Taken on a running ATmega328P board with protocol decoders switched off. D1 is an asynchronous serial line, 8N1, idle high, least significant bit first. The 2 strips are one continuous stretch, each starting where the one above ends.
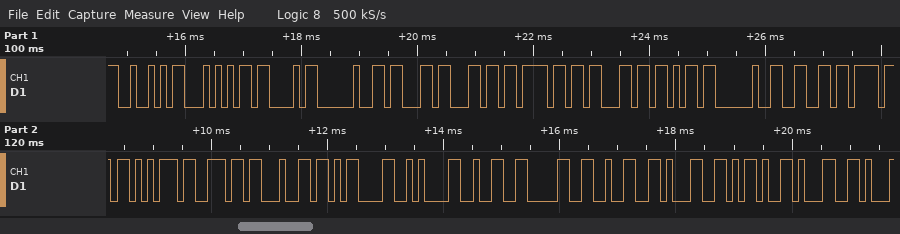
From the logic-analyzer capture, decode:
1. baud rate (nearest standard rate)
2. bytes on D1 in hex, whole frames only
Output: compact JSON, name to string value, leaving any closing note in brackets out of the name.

{"baud rate": "9600 baud", "bytes on D1 in hex, whole frames only": "0x52 0x54 0x43 0x20 0x63 0x6C 0x6F 0x63 0x6B 0x20 0x66 0x6F 0x75 0x6E 0x64 0x0D 0x0A 0x32 0x30 0x32 0x31 0x2D 0x31"}
